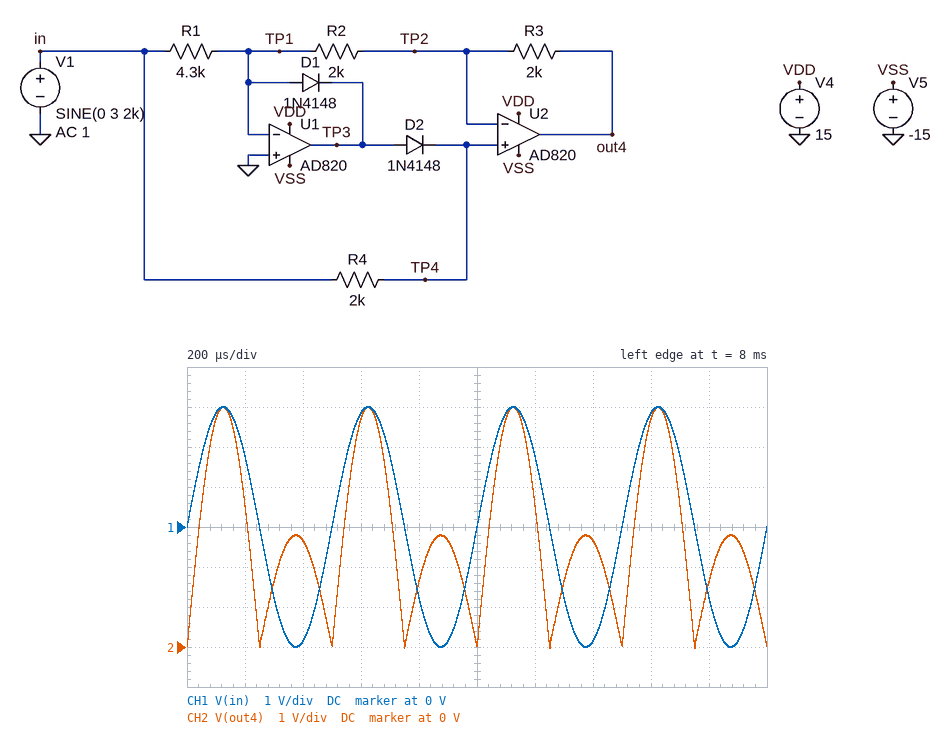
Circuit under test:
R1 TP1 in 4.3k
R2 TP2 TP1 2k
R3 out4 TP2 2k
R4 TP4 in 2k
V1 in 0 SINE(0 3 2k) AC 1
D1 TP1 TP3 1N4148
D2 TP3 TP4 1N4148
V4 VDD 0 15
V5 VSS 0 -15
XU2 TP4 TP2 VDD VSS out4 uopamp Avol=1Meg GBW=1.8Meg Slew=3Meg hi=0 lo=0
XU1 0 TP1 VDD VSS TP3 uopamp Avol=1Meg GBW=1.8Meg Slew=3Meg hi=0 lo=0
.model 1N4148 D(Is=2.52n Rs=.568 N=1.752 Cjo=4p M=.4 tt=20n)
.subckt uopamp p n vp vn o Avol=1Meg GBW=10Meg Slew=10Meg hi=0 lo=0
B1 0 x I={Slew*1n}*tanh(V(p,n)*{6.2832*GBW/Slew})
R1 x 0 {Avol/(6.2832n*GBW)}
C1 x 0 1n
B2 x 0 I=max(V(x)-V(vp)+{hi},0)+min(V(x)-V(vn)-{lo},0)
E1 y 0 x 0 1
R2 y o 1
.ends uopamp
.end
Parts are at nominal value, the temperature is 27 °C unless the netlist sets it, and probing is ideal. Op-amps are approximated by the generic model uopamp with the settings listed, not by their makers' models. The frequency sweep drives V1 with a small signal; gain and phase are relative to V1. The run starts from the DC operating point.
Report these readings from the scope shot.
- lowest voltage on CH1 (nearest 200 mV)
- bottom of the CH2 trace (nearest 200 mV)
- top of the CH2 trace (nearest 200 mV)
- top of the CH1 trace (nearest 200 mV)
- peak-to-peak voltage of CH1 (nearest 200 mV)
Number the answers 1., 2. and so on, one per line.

1. -3.0 V
2. 0 V
3. 6.0 V
4. 3.0 V
5. 6.0 V
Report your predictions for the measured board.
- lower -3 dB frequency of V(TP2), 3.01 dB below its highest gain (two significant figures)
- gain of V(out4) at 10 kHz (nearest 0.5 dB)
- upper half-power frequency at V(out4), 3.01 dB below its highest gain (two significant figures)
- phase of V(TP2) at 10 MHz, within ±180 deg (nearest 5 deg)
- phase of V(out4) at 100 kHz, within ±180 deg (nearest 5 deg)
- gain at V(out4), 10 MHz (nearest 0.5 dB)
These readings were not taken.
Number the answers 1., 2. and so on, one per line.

1. 220 Hz
2. -0.5 dB
3. 1.4 MHz
4. -50 deg
5. -5 deg
6. -18.5 dB
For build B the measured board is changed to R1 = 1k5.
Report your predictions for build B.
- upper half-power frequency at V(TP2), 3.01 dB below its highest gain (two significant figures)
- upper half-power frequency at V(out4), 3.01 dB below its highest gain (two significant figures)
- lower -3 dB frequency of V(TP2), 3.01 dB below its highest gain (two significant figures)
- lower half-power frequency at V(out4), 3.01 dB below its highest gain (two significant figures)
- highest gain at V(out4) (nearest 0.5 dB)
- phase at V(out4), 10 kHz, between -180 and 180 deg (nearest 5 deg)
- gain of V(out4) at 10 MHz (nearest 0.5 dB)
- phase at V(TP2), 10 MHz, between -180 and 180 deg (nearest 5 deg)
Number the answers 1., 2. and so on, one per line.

1. 1.4 MHz
2. 1.2 MHz
3. 160 Hz
4. 140 Hz
5. -1.0 dB
6. 0 deg
7. -20.5 dB
8. -25 deg
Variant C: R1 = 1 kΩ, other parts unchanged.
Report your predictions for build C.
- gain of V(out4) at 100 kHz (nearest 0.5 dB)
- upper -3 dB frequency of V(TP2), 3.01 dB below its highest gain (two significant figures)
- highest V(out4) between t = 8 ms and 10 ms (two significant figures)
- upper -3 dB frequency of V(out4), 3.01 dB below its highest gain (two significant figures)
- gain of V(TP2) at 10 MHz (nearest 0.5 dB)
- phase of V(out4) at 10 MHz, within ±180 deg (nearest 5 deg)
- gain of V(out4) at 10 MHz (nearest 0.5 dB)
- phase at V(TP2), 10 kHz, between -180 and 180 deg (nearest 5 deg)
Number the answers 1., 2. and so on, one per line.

1. -1.0 dB
2. 1.3 MHz
3. 12 V
4. 900 kHz
5. -9.0 dB
6. -120 deg
7. -21.5 dB
8. 0 deg
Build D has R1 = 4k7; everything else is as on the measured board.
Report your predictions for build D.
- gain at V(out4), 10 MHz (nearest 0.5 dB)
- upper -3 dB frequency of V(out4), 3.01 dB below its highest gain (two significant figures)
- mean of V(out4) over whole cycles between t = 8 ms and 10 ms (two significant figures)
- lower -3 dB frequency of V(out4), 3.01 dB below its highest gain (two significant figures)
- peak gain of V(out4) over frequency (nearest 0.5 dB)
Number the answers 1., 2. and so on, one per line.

1. -18.0 dB
2. 1.5 MHz
3. 2.7 V
4. 130 Hz
5. -0.5 dB
